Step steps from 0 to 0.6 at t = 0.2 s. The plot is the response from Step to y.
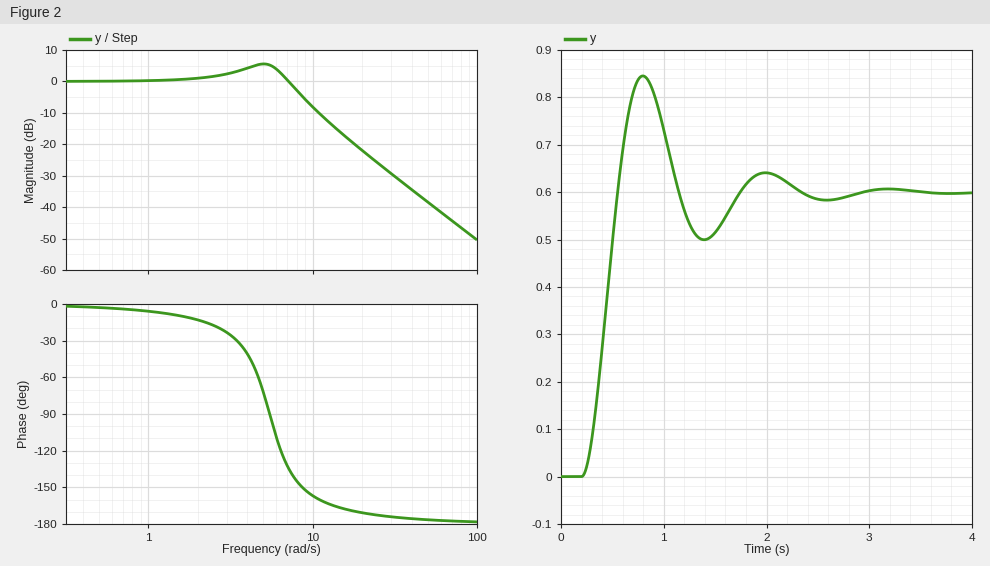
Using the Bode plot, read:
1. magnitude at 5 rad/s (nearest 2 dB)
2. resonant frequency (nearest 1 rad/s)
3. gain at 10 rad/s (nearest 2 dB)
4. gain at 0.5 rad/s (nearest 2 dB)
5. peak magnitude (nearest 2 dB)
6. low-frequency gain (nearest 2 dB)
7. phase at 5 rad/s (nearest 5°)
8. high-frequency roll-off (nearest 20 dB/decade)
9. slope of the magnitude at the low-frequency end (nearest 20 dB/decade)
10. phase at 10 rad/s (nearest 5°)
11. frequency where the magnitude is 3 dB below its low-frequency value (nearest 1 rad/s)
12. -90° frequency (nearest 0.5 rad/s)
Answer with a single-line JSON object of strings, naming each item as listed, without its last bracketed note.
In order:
{"magnitude at 5 rad/s": "6 dB", "resonant frequency": "5 rad/s", "gain at 10 rad/s": "-8 dB", "gain at 0.5 rad/s": "0 dB", "peak magnitude": "6 dB", "low-frequency gain": "0 dB", "phase at 5 rad/s": "-70°", "high-frequency roll-off": "-40 dB/decade", "slope of the magnitude at the low-frequency end": "0 dB/decade", "phase at 10 rad/s": "-155°", "frequency where the magnitude is 3 dB below its low-frequency value": "8 rad/s", "-90° frequency": "5.5 rad/s"}
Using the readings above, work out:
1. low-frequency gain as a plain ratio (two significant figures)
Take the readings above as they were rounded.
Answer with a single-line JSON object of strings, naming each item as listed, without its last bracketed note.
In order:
{"low-frequency gain as a plain ratio": "1.0"}
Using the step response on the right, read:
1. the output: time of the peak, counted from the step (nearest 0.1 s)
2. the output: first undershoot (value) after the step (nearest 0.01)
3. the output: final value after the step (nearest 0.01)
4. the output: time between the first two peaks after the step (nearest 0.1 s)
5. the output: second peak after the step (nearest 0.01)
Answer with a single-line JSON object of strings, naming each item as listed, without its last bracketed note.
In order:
{"the output: time of the peak, counted from the step": "0.6 s", "the output: first undershoot (value) after the step": "0.50", "the output: final value after the step": "0.60", "the output: time between the first two peaks after the step": "1.2 s", "the output: second peak after the step": "0.64"}
